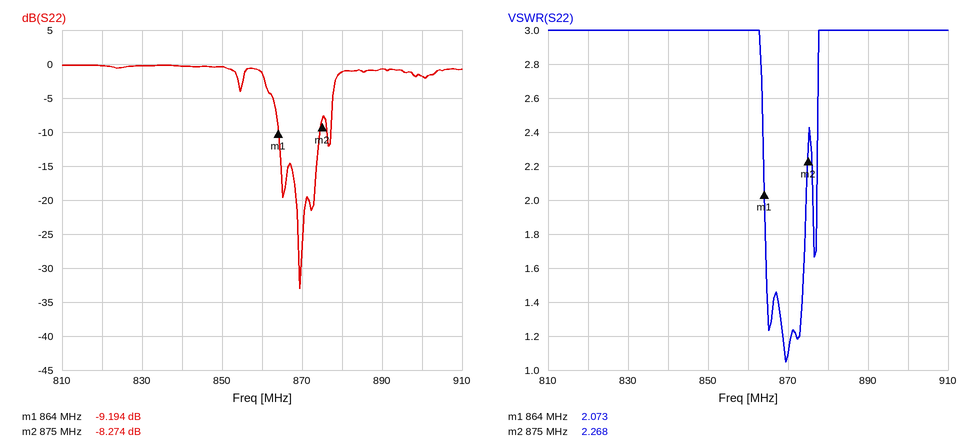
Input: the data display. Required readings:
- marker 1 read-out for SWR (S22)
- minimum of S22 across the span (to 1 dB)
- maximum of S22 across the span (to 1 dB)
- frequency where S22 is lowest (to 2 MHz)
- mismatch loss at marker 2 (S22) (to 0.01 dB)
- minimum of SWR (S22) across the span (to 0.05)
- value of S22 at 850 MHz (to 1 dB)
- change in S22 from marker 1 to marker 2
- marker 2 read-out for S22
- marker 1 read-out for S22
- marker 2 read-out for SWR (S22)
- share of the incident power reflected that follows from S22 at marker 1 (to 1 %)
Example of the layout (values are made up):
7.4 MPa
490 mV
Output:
2.073
-33 dB
0 dB
870 MHz
0.70 dB
1.05
0 dB
0.920 dB
-8.274 dB
-9.194 dB
2.268
12 %
